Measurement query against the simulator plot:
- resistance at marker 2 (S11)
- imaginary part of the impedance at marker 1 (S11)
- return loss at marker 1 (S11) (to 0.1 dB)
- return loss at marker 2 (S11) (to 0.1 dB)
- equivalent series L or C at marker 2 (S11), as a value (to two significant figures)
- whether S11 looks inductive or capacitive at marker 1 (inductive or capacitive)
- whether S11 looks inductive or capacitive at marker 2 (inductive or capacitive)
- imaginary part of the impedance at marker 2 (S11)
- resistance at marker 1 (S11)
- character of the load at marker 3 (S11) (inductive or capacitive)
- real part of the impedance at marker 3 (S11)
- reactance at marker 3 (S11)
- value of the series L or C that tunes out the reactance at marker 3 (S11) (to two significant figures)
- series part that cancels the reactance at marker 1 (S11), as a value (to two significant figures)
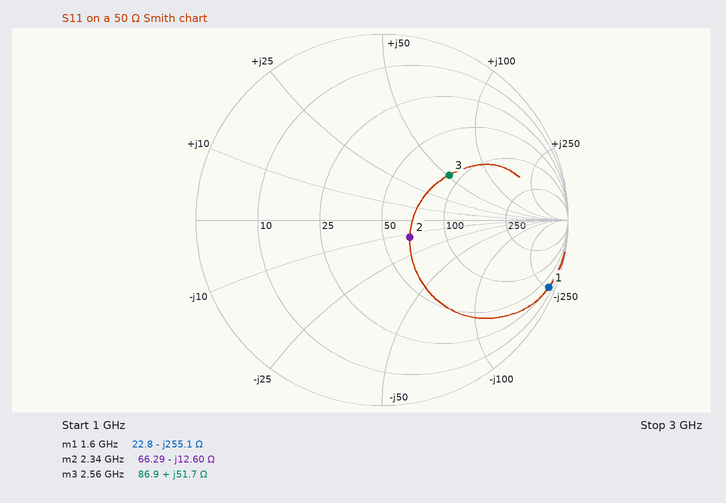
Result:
66.29 Ω
-255.1 Ω
0.3 dB
15.1 dB
5.4 pF
capacitive
capacitive
-12.60 Ω
22.8 Ω
inductive
86.9 Ω
+51.7 Ω
1.2 pF
25 nH
